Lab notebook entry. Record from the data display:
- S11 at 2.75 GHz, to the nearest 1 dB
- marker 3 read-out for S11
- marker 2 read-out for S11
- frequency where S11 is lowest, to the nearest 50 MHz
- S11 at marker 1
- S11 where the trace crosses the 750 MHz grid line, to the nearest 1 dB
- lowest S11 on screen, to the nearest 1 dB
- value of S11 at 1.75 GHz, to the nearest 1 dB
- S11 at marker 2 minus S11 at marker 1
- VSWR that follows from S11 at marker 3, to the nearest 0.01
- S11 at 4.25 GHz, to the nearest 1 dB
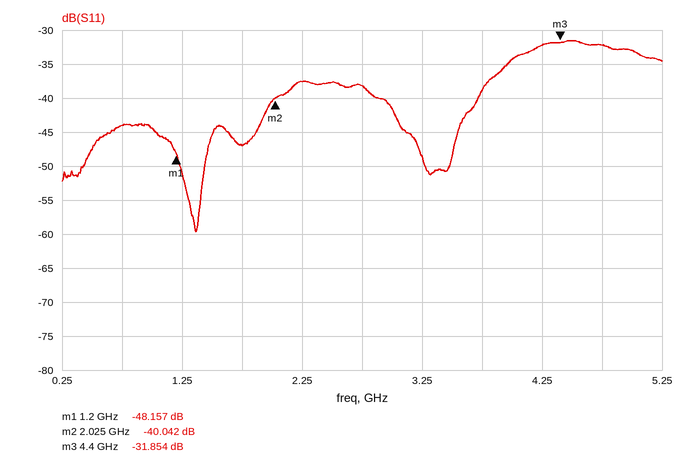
-38 dB
-31.854 dB
-40.042 dB
1.35 GHz
-48.157 dB
-44 dB
-60 dB
-47 dB
8.115 dB
1.05
-32 dB
